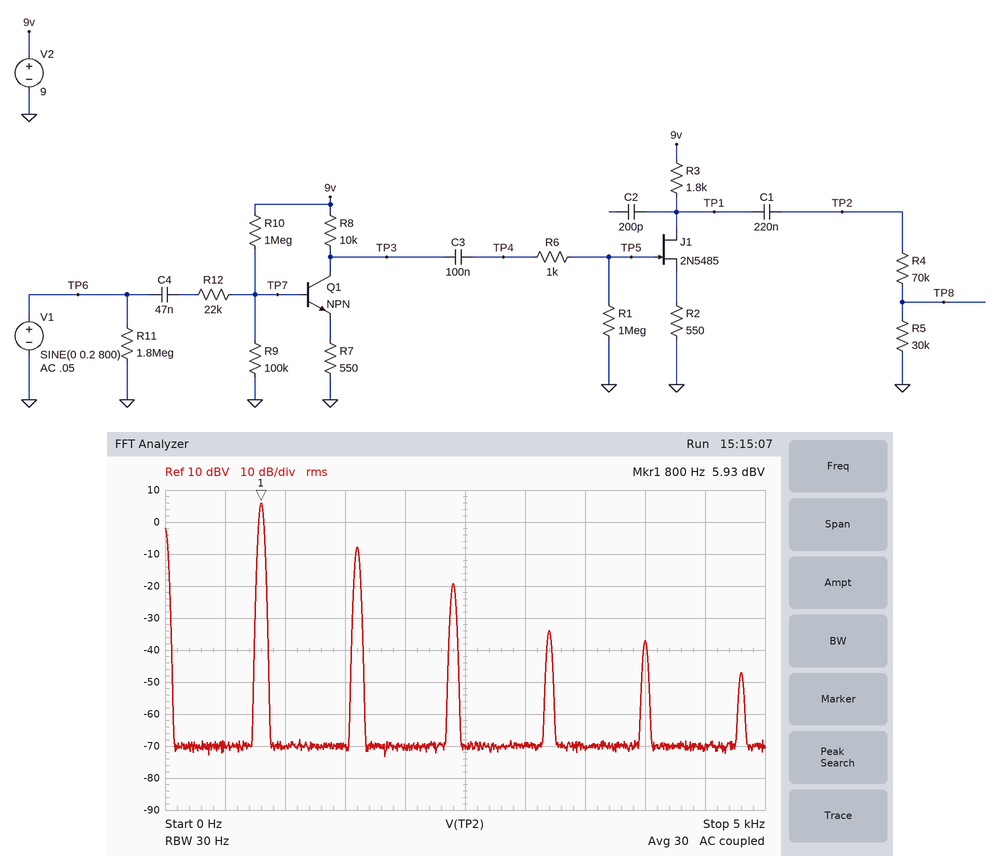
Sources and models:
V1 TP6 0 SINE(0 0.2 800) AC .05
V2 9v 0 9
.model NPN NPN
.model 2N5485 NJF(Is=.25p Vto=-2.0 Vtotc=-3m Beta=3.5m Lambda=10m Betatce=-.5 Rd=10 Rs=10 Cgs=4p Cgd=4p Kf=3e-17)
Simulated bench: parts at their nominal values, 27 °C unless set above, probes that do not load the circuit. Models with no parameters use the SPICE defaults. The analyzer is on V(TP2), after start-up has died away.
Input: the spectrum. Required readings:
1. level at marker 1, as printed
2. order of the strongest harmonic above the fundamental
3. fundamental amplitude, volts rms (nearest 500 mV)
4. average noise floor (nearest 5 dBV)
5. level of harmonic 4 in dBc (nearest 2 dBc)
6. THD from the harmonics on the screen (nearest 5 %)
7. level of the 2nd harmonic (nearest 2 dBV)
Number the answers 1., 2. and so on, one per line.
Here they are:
1. 5.93 dBV
2. 2
3. 2.0 V
4. -70 dBV
5. -40 dBc
6. 20 %
7. -8 dBV
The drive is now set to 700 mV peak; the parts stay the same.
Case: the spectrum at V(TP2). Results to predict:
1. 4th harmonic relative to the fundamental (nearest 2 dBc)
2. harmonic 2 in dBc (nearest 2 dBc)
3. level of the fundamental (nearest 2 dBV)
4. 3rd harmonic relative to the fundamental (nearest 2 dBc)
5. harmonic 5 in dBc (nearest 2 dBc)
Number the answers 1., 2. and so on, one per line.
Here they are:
1. -12 dBc
2. -8 dBc
3. 8 dBV
4. -20 dBc
5. -22 dBc
